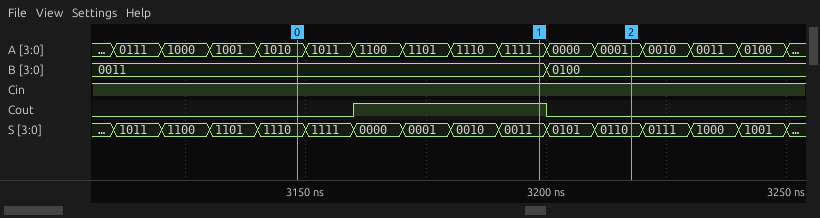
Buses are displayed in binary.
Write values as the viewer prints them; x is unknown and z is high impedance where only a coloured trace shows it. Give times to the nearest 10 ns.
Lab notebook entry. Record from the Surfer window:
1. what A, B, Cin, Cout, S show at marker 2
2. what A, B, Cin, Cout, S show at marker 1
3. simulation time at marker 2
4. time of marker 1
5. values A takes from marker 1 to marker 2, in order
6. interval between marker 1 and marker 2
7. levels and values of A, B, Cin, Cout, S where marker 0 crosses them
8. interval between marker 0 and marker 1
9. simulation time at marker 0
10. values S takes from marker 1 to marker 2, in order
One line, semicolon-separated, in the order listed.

A=0001, B=0100, Cin=1, Cout=0, S=0110; A=1111, B=0011, Cin=1, Cout=1, S=0011; 3220 ns; 3200 ns; 1111, 0000, 0001; 20 ns; A=1010, B=0011, Cin=1, Cout=0, S=1110; 50 ns; 3150 ns; 0011, 0101, 0110
